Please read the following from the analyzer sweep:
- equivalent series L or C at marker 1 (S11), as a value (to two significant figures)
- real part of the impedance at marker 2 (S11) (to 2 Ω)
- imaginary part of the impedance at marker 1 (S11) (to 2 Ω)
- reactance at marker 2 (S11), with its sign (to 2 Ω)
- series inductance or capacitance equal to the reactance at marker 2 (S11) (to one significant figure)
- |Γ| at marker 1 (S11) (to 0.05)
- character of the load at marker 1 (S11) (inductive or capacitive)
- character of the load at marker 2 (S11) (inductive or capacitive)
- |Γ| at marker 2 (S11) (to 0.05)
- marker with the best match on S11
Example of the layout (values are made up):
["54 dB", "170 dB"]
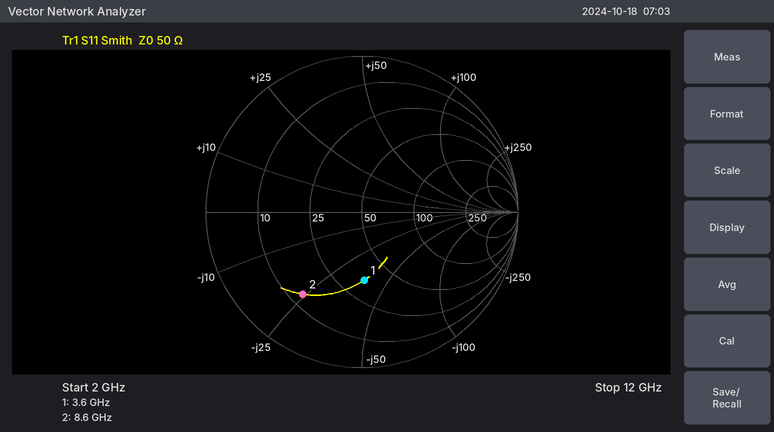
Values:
["1.2 pF", "14 Ω", "-38 Ω", "-24 Ω", "800 fF", "0.45", "capacitive", "capacitive", "0.65", "marker 1"]
